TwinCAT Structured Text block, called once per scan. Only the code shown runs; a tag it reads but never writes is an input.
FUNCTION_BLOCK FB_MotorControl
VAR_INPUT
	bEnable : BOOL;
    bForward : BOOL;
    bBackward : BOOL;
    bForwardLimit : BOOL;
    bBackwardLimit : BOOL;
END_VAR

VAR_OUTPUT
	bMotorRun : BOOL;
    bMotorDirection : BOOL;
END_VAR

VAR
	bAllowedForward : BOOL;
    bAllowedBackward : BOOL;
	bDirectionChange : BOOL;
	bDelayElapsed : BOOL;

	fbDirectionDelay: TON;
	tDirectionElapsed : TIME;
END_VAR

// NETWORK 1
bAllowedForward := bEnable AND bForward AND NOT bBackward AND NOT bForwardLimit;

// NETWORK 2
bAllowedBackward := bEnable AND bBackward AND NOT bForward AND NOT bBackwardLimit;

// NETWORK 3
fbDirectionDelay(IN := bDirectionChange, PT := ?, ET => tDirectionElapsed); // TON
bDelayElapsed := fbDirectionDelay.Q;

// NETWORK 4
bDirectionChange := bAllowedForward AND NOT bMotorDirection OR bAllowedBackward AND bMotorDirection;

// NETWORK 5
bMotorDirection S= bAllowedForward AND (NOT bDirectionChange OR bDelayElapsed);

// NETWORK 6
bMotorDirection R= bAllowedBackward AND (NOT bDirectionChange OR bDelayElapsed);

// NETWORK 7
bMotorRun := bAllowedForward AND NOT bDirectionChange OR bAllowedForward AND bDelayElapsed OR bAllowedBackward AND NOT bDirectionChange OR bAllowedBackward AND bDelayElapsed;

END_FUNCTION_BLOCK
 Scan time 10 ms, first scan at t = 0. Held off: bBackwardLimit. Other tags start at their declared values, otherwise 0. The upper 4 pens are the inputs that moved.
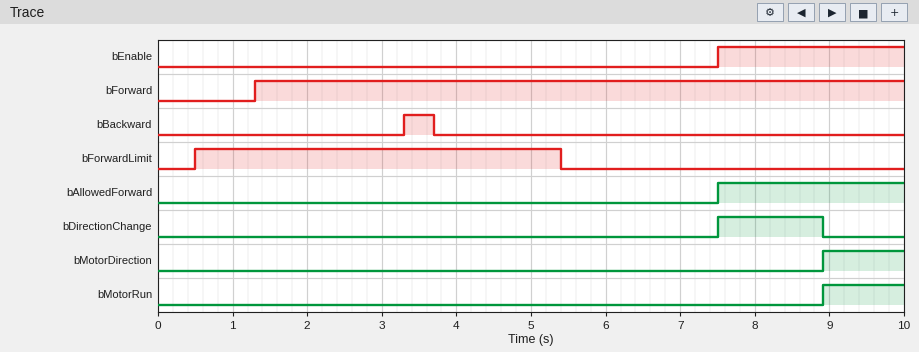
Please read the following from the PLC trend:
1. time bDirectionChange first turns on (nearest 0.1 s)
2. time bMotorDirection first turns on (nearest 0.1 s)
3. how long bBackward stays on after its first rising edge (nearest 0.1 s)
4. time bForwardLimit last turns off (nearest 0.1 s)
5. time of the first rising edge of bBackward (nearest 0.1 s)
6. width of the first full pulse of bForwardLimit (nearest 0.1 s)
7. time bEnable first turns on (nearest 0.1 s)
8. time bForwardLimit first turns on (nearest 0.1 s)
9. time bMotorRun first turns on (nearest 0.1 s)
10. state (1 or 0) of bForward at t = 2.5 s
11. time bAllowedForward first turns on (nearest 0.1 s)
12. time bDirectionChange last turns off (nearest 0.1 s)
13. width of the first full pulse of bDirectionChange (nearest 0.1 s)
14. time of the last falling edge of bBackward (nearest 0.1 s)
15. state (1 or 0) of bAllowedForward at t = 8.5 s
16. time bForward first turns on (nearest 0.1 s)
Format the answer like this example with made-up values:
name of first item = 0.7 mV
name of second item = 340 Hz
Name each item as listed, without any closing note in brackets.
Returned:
time bDirectionChange first turns on = 7.5 s
time bMotorDirection first turns on = 8.9 s
how long bBackward stays on after its first rising edge = 0.4 s
time bForwardLimit last turns off = 5.4 s
time of the first rising edge of bBackward = 3.3 s
width of the first full pulse of bForwardLimit = 4.9 s
time bEnable first turns on = 7.5 s
time bForwardLimit first turns on = 0.5 s
time bMotorRun first turns on = 8.9 s
state (1 or 0) of bForward at t = 2.5 s = 1
time bAllowedForward first turns on = 7.5 s
time bDirectionChange last turns off = 8.9 s
width of the first full pulse of bDirectionChange = 1.4 s
time of the last falling edge of bBackward = 3.7 s
state (1 or 0) of bAllowedForward at t = 8.5 s = 1
time bForward first turns on = 1.3 s
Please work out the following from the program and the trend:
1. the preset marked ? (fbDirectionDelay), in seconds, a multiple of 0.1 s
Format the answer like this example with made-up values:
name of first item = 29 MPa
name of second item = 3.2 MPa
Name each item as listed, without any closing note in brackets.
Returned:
the preset marked ? (fbDirectionDelay), in seconds, a multiple of 0.1 s = 1.4 s
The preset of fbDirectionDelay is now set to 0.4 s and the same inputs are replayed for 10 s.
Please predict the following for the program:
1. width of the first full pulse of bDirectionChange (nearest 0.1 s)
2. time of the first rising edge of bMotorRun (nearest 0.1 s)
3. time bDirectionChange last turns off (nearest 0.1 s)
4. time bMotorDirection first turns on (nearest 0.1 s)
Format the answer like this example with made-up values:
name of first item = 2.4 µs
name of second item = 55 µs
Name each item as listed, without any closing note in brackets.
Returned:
width of the first full pulse of bDirectionChange = 0.4 s
time of the first rising edge of bMotorRun = 7.9 s
time bDirectionChange last turns off = 7.9 s
time bMotorDirection first turns on = 7.9 s
